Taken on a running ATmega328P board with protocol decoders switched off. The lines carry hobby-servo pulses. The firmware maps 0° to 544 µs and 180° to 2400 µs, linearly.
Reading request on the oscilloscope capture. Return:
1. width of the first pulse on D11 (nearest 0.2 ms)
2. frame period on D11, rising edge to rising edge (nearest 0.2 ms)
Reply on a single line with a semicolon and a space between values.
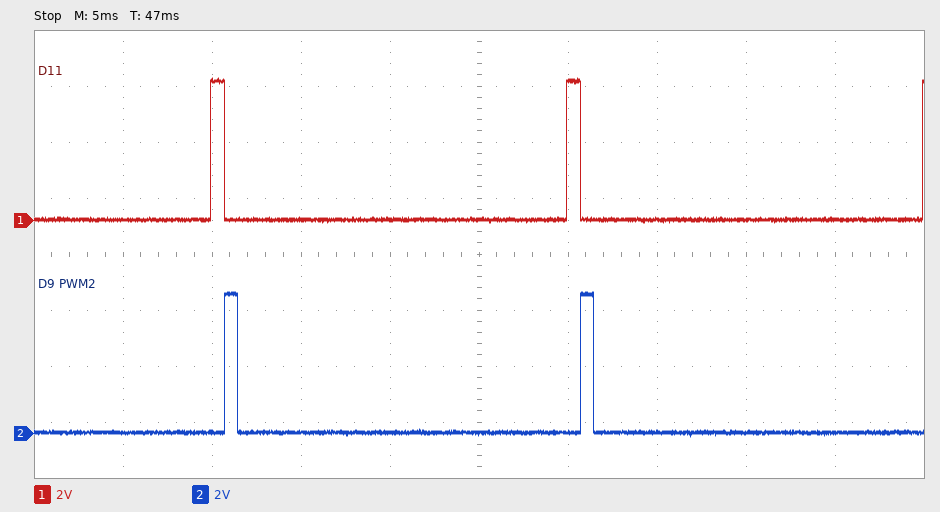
0.8 ms; 20.0 ms
